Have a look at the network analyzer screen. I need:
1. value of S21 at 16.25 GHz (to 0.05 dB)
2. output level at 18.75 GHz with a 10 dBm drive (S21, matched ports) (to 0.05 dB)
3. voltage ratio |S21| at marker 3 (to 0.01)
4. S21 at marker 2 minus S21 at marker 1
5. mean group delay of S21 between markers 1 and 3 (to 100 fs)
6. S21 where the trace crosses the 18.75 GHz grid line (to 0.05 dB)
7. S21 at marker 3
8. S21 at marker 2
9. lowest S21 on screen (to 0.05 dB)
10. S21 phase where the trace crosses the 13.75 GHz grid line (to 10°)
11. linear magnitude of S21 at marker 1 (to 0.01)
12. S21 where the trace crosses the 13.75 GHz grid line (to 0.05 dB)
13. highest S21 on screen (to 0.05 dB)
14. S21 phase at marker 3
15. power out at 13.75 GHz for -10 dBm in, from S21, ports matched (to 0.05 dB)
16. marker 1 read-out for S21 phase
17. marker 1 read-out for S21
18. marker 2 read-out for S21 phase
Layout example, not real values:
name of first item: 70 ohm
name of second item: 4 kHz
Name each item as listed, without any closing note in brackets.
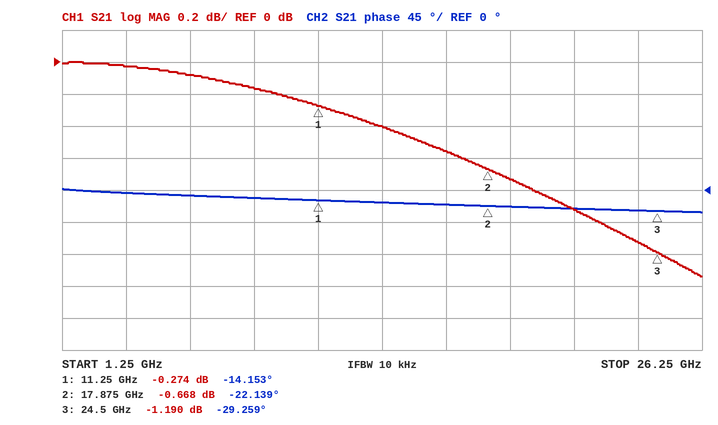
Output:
value of S21 at 16.25 GHz: -0.55 dB
output level at 18.75 GHz with a 10 dBm drive (S21, matched ports): 9.25 dBm
voltage ratio |S21| at marker 3: 0.87
S21 at marker 2 minus S21 at marker 1: -0.394 dB
mean group delay of S21 between markers 1 and 3: 3.2 ps
S21 where the trace crosses the 18.75 GHz grid line: -0.75 dB
S21 at marker 3: -1.190 dB
S21 at marker 2: -0.668 dB
lowest S21 on screen: -1.35 dB
S21 phase where the trace crosses the 13.75 GHz grid line: -20°
linear magnitude of S21 at marker 1: 0.97
S21 where the trace crosses the 13.75 GHz grid line: -0.40 dB
highest S21 on screen: 0.00 dB
S21 phase at marker 3: -29.259°
power out at 13.75 GHz for -10 dBm in, from S21, ports matched: -10.40 dBm
marker 1 read-out for S21 phase: -14.153°
marker 1 read-out for S21: -0.274 dB
marker 2 read-out for S21 phase: -22.139°
